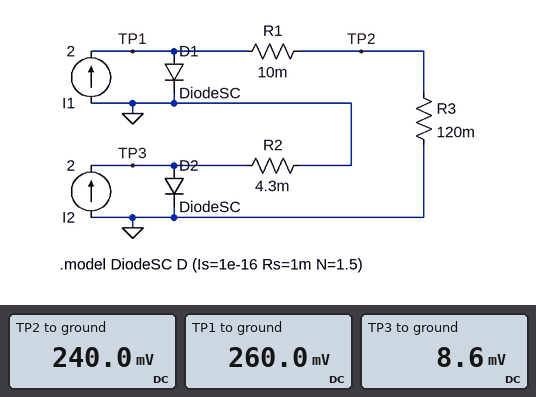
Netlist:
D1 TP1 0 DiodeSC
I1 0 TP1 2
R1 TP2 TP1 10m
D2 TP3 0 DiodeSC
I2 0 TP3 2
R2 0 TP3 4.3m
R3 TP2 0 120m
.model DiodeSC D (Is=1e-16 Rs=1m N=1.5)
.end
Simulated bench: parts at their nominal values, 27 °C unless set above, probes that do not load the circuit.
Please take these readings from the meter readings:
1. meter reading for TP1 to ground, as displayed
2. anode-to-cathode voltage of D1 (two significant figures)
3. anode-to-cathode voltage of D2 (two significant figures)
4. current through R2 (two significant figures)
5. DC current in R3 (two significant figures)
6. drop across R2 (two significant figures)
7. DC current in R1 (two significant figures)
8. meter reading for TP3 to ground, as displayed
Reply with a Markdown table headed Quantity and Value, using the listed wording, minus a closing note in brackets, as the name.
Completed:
| Quantity | Value |
|---|---|
| meter reading for TP1 to ground, as displayed | 260.0 mV |
| anode-to-cathode voltage of D1 | 260 mV |
| anode-to-cathode voltage of D2 | 8.6 mV |
| current through R2 | 2.0 A |
| DC current in R3 | 2.0 A |
| drop across R2 | 8.6 mV |
| DC current in R1 | 2.0 A |
| meter reading for TP3 to ground, as displayed | 8.6 mV |
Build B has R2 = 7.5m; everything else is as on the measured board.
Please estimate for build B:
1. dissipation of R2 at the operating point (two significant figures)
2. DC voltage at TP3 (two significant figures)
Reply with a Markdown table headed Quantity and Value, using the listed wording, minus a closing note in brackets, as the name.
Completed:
| Quantity | Value |
|---|---|
| dissipation of R2 at the operating point | 30 mW |
| DC voltage at TP3 | 15 mV |
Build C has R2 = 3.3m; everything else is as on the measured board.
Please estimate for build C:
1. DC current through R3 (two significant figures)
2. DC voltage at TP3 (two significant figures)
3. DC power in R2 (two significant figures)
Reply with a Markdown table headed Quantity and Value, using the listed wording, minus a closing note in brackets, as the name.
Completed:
| Quantity | Value |
|---|---|
| DC current through R3 | 2.0 A |
| DC voltage at TP3 | 6.6 mV |
| DC power in R2 | 13 mW |
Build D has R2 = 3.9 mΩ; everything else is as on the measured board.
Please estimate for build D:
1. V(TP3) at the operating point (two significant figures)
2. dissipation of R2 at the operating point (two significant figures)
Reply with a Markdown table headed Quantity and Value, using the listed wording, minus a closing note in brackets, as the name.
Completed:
| Quantity | Value |
|---|---|
| V(TP3) at the operating point | 7.8 mV |
| dissipation of R2 at the operating point | 16 mW |
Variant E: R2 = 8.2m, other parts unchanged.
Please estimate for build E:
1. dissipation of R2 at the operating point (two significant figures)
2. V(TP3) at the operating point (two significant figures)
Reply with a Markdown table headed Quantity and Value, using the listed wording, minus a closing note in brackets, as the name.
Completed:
| Quantity | Value |
|---|---|
| dissipation of R2 at the operating point | 33 mW |
| V(TP3) at the operating point | 16 mV |
